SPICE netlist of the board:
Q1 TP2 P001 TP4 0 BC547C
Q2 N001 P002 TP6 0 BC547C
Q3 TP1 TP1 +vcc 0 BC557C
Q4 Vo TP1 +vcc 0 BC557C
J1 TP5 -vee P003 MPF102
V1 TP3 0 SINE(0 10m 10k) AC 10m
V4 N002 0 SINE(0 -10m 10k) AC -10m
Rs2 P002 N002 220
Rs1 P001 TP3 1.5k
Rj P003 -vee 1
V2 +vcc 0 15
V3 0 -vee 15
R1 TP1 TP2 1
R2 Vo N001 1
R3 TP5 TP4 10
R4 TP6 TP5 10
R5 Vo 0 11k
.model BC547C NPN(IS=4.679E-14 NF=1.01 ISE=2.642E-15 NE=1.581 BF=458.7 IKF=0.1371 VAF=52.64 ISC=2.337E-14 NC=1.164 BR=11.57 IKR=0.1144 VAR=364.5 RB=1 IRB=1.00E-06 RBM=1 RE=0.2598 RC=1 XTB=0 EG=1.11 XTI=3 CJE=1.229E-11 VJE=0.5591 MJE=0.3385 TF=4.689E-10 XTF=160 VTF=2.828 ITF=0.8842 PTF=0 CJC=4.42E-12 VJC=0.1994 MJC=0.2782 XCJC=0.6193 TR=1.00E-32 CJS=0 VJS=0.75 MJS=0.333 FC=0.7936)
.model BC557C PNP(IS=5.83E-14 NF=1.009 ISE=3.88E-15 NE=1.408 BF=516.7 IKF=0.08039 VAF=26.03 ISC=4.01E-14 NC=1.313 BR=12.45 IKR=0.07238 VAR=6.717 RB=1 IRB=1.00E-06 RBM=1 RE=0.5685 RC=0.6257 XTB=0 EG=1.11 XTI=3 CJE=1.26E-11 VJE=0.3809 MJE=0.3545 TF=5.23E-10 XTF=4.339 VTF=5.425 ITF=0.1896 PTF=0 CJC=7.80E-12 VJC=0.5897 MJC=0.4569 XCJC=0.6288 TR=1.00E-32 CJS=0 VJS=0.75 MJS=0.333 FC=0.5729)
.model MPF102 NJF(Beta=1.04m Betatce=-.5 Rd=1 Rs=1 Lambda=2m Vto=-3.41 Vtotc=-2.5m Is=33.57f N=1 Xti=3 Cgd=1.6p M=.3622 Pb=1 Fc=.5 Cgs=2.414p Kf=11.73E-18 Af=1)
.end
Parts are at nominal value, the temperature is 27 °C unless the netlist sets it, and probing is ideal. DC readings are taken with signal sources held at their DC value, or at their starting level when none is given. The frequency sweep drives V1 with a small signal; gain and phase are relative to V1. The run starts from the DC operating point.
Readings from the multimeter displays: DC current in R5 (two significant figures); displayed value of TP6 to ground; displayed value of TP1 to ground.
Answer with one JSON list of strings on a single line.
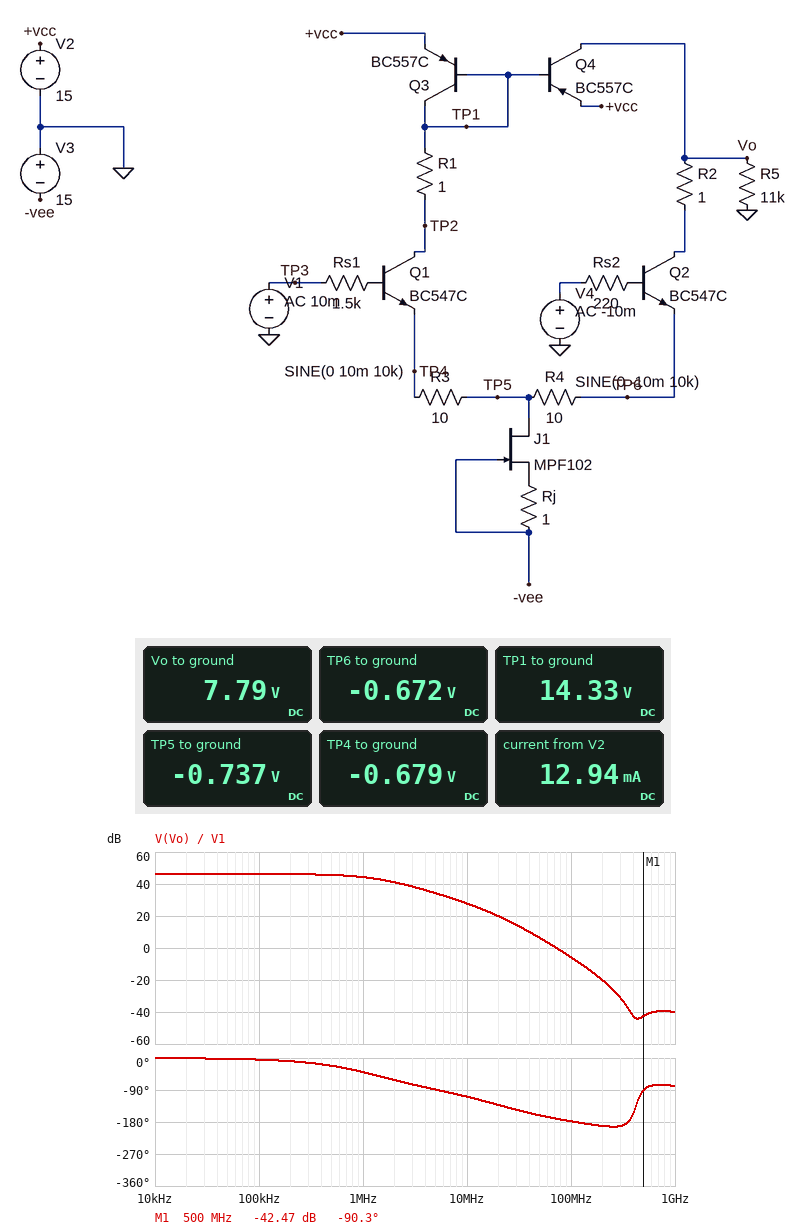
["710 µA", "-0.672 V", "14.33 V"]
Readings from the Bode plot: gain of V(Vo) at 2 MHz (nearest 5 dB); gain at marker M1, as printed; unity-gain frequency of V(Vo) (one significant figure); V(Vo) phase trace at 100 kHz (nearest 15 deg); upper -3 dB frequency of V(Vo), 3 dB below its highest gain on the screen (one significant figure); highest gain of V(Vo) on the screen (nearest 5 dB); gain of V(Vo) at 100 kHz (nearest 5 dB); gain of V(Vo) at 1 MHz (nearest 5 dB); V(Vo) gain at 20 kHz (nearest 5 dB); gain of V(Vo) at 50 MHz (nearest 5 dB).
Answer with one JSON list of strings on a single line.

["40 dB", "-42.47 dB", "70 MHz", "0 deg", "1 MHz", "45 dB", "45 dB", "45 dB", "45 dB", "5 dB"]
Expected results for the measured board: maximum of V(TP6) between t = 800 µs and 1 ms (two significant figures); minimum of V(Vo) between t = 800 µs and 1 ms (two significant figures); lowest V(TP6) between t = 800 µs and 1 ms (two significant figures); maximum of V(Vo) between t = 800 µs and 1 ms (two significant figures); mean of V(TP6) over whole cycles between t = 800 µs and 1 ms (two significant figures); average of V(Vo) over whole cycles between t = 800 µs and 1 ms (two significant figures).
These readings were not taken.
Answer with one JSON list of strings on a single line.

["-670 mV", "3.5 V", "-680 mV", "12 V", "-670 mV", "7.7 V"]
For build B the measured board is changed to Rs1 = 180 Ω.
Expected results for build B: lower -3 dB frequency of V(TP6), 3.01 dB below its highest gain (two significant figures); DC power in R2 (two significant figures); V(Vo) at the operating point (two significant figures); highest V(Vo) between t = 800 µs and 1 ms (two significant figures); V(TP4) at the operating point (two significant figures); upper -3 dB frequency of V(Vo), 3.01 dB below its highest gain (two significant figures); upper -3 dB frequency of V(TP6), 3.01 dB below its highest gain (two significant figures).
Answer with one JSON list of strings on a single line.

["1.4 MHz", "37 µW", "11 V", "14 V", "-670 mV", "1.7 MHz", "150 MHz"]
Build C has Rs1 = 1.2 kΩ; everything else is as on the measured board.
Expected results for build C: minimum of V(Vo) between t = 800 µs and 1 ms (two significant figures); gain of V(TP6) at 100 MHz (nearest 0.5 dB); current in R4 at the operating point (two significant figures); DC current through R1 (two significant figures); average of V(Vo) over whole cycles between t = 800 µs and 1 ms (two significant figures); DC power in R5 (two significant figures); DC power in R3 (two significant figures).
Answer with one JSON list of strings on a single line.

["4.1 V", "-15.0 dB", "6.4 mA", "5.9 mA", "8.3 V", "6.4 mW", "350 µW"]
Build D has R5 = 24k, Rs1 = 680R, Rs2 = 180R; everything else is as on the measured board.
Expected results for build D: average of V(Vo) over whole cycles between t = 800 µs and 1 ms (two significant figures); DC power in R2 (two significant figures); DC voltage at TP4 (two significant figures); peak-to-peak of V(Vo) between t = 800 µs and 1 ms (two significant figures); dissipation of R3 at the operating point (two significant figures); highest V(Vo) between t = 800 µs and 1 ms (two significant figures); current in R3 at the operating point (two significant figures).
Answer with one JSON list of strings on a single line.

["11 V", "39 µW", "-670 mV", "8.8 V", "360 µW", "15 V", "6.0 mA"]
